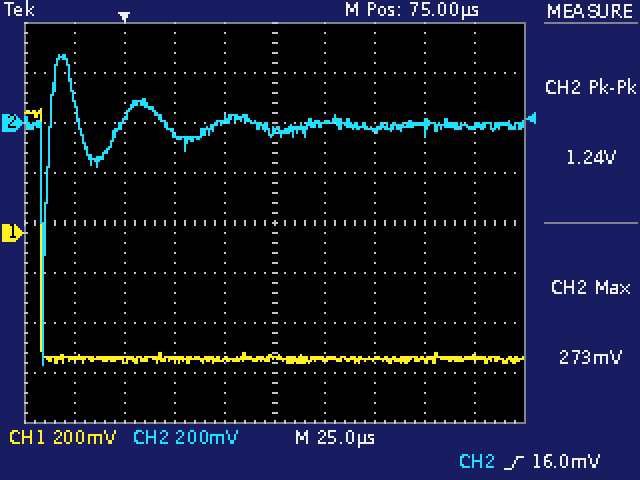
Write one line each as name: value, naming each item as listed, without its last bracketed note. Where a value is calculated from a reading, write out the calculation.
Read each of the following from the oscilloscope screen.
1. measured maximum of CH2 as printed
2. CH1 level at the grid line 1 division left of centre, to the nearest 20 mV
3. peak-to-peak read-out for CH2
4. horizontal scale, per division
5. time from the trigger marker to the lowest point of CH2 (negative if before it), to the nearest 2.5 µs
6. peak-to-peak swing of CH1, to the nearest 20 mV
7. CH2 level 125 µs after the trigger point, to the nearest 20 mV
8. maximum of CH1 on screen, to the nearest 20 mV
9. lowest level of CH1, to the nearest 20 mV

measured maximum of CH2 as printed: 273 mV
CH1 level at the grid line 1 division left of centre, to the nearest 20 mV: -500 mV
peak-to-peak read-out for CH2: 1.24 V
horizontal scale, per division: 25 µs
time from the trigger marker to the lowest point of CH2 (negative if before it), to the nearest 2.5 µs: -40.0 µs
peak-to-peak swing of CH1, to the nearest 20 mV: 500 mV − (-520 mV) = 1.02 V
CH2 level 125 µs after the trigger point, to the nearest 20 mV: -20 mV
maximum of CH1 on screen, to the nearest 20 mV: 500 mV
lowest level of CH1, to the nearest 20 mV: -520 mV
